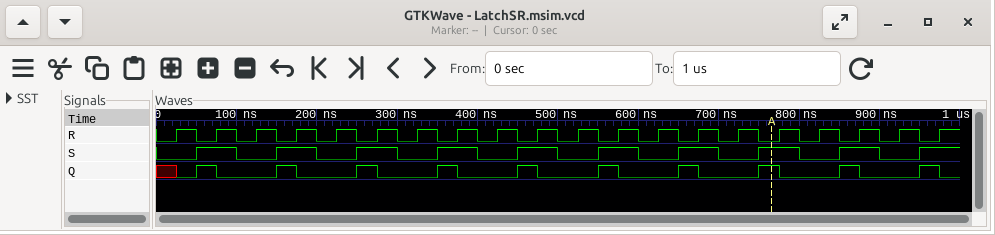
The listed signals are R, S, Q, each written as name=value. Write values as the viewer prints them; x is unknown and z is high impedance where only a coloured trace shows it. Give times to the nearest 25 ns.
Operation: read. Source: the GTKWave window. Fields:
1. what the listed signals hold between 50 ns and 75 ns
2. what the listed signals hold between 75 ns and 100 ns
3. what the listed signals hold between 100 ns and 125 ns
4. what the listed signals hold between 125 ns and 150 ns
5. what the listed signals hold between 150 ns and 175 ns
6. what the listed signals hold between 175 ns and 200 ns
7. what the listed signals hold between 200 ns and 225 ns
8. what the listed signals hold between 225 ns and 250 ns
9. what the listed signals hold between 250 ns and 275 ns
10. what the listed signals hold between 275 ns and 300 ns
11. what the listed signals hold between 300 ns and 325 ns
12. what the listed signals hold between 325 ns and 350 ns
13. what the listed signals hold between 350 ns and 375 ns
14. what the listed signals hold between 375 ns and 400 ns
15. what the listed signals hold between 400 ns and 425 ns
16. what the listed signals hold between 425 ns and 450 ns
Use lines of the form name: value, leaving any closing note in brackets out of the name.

what the listed signals hold between 50 ns and 75 ns: R=0, S=1, Q=1
what the listed signals hold between 75 ns and 100 ns: R=1, S=1, Q=0
what the listed signals hold between 100 ns and 125 ns: R=0, S=0, Q=0
what the listed signals hold between 125 ns and 150 ns: R=1, S=0, Q=0
what the listed signals hold between 150 ns and 175 ns: R=0, S=1, Q=1
what the listed signals hold between 175 ns and 200 ns: R=1, S=1, Q=0
what the listed signals hold between 200 ns and 225 ns: R=0, S=0, Q=0
what the listed signals hold between 225 ns and 250 ns: R=1, S=0, Q=0
what the listed signals hold between 250 ns and 275 ns: R=0, S=1, Q=1
what the listed signals hold between 275 ns and 300 ns: R=1, S=1, Q=0
what the listed signals hold between 300 ns and 325 ns: R=0, S=0, Q=0
what the listed signals hold between 325 ns and 350 ns: R=1, S=0, Q=0
what the listed signals hold between 350 ns and 375 ns: R=0, S=1, Q=1
what the listed signals hold between 375 ns and 400 ns: R=1, S=1, Q=0
what the listed signals hold between 400 ns and 425 ns: R=0, S=0, Q=0
what the listed signals hold between 425 ns and 450 ns: R=1, S=0, Q=0
